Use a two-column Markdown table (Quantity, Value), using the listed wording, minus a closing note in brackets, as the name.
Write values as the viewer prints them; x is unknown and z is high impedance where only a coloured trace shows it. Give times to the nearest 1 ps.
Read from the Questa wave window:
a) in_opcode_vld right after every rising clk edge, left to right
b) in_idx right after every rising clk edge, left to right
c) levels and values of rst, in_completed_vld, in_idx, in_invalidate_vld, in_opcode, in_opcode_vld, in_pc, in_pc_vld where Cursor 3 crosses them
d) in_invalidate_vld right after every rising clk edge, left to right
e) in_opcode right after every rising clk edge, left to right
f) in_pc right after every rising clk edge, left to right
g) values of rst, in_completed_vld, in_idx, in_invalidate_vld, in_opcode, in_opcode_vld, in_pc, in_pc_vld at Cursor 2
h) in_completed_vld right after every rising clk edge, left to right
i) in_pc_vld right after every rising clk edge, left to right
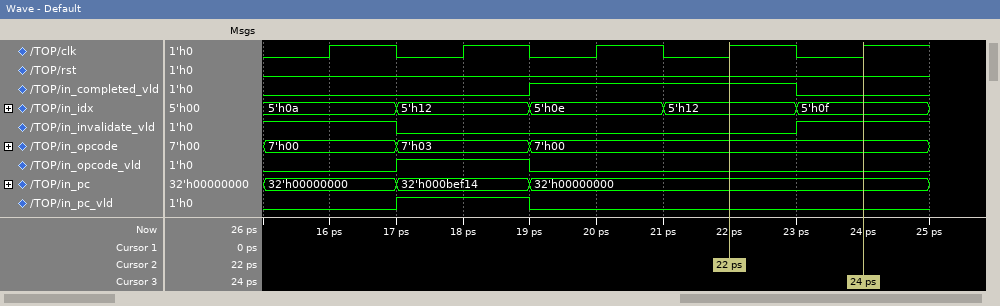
| Quantity | Value |
|---|---|
| in_opcode_vld right after every rising clk edge, left to right | 0 1 0 0 0 |
| in_idx right after every rising clk edge, left to right | 5'h0a, 5'h12, 5'h0e, 5'h12, 5'h0f |
| levels and values of rst, in_completed_vld, in_idx, in_invalidate_vld, in_opcode, in_opcode_vld, in_pc, in_pc_vld where Cursor 3 crosses them | rst=0, in_completed_vld=0, in_idx=5'h0f, in_invalidate_vld=1, in_opcode=7'h00, in_opcode_vld=0, in_pc=32'h00000000, in_pc_vld=0 |
| in_invalidate_vld right after every rising clk edge, left to right | 1 0 0 0 1 |
| in_opcode right after every rising clk edge, left to right | 7'h00, 7'h03, 7'h00, 7'h00, 7'h00 |
| in_pc right after every rising clk edge, left to right | 32'h00000000, 32'h000bef14, 32'h00000000, 32'h00000000, 32'h00000000 |
| values of rst, in_completed_vld, in_idx, in_invalidate_vld, in_opcode, in_opcode_vld, in_pc, in_pc_vld at Cursor 2 | rst=0, in_completed_vld=1, in_idx=5'h12, in_invalidate_vld=0, in_opcode=7'h00, in_opcode_vld=0, in_pc=32'h00000000, in_pc_vld=0 |
| in_completed_vld right after every rising clk edge, left to right | 0 0 1 1 0 |
| in_pc_vld right after every rising clk edge, left to right | 0 1 0 0 0 |
